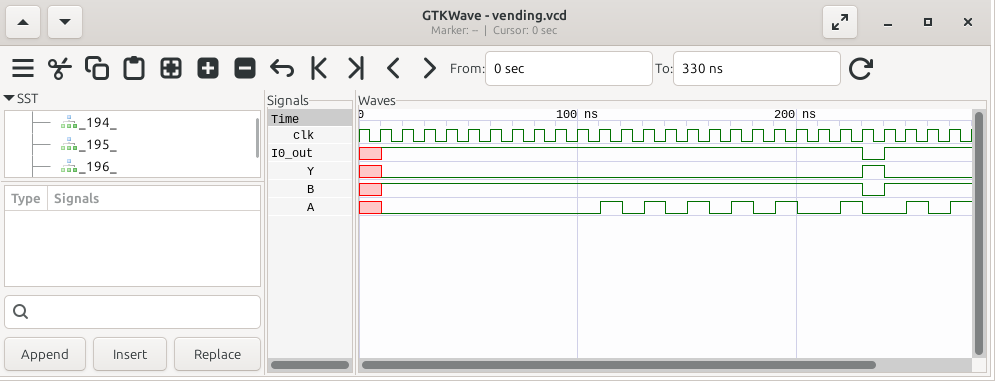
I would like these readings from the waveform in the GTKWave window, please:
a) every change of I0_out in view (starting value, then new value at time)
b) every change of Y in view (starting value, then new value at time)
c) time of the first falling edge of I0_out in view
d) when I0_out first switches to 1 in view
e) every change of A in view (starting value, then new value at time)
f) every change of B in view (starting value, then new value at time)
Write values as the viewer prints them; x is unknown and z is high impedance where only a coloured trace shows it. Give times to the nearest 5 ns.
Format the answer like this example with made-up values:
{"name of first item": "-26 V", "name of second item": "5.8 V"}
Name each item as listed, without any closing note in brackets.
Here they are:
{"every change of I0_out in view": "x, 1 at 10 ns, 0 at 230 ns, 1 at 240 ns", "every change of Y in view": "x, 0 at 10 ns, 1 at 230 ns, 0 at 240 ns", "time of the first falling edge of I0_out in view": "230 ns", "when I0_out first switches to 1 in view": "10 ns", "every change of A in view": "x, 0 at 10 ns, 1 at 110 ns, 0 at 120 ns, 1 at 130 ns, 0 at 140 ns, 1 at 150 ns, 0 at 160 ns, 1 at 170 ns, 0 at 180 ns, 1 at 190 ns, 0 at 200 ns, 1 at 220 ns, 0 at 230 ns, 1 at 250 ns, 0 at 260 ns, 1 at 270 ns", "every change of B in view": "x, 1 at 10 ns, 0 at 230 ns, 1 at 240 ns"}
